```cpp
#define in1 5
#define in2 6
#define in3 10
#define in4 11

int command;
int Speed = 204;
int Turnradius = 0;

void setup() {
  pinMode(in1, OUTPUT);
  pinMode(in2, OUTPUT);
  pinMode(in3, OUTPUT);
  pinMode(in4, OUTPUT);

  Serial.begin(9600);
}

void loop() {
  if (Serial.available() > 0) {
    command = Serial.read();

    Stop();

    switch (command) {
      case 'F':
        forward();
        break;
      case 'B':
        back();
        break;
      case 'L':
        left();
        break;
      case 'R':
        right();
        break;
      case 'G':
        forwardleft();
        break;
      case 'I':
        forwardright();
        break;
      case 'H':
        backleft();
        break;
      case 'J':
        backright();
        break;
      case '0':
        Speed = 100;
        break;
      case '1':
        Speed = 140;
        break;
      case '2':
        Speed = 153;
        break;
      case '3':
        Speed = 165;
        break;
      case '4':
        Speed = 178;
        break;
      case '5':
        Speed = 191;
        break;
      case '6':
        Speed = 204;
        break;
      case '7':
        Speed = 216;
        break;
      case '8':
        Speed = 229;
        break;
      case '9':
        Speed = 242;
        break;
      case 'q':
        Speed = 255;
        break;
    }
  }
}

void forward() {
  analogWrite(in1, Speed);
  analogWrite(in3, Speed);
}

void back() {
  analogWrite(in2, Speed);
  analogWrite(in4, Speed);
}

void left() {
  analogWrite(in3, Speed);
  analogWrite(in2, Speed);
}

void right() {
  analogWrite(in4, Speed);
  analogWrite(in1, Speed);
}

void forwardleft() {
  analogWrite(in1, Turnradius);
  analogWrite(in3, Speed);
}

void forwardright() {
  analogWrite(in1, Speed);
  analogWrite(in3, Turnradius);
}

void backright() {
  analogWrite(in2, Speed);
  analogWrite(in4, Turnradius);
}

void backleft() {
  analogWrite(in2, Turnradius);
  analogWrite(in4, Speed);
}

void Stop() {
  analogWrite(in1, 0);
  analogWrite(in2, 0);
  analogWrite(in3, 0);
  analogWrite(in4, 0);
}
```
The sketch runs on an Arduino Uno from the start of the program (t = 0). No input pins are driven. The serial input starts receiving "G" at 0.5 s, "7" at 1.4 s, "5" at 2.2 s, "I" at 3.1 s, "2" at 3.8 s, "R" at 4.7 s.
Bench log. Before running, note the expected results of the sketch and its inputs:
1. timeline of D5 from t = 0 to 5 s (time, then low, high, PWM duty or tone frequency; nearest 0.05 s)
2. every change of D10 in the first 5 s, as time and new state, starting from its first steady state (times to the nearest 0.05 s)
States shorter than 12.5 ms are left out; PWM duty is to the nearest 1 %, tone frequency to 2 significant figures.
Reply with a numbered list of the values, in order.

1. 0 s low; 3.1 s PWM 75 %; 3.8 s low; 4.7 s PWM 60 %
2. 0 s low; 0.5 s PWM 80 %; 1.4 s low
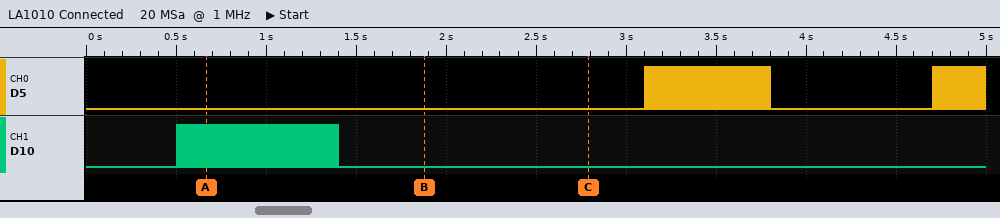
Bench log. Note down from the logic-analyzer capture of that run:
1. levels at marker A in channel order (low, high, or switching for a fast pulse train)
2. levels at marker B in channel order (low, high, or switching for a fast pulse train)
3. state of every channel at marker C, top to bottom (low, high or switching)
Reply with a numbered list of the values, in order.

1. D5 low, D10 switching
2. D5 low, D10 low
3. D5 low, D10 low
